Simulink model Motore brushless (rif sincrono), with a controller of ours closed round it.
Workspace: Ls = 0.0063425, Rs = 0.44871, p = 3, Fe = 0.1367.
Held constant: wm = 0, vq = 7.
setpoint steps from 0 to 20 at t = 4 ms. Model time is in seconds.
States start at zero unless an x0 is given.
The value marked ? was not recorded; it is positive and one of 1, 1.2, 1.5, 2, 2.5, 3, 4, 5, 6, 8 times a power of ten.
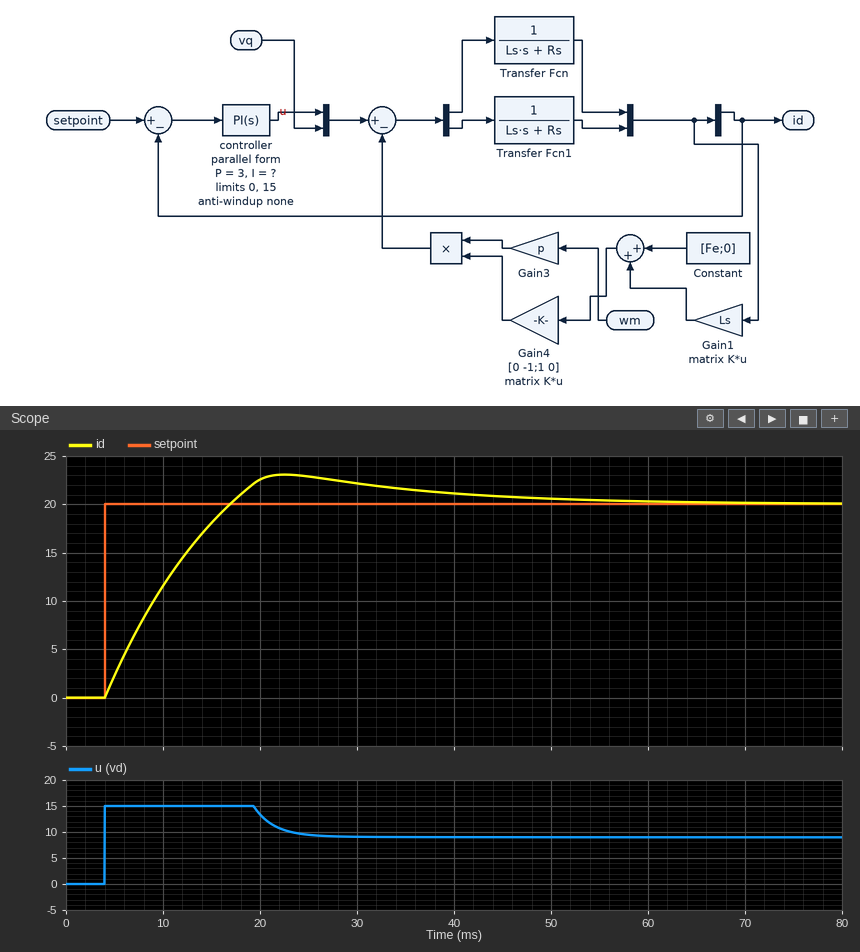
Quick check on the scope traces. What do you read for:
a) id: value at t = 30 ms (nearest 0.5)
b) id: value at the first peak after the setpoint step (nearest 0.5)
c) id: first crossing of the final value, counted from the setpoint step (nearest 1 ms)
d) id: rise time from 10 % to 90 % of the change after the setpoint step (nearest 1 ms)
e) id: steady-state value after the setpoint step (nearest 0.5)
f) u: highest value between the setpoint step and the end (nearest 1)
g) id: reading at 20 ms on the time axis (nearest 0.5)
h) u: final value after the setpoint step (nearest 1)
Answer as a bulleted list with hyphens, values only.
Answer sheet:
- 22.0
- 23.0
- 13 ms
- 10 ms
- 20.0
- 15
- 22.5
- 9
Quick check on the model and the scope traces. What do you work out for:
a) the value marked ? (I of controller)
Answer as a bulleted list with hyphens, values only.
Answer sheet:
- 200
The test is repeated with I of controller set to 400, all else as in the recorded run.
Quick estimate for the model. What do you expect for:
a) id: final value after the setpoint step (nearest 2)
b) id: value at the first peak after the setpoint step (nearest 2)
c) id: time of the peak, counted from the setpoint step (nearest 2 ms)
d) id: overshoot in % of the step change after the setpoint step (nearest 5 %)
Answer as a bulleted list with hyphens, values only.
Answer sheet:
- 20
- 26
- 22 ms
- 30 %
